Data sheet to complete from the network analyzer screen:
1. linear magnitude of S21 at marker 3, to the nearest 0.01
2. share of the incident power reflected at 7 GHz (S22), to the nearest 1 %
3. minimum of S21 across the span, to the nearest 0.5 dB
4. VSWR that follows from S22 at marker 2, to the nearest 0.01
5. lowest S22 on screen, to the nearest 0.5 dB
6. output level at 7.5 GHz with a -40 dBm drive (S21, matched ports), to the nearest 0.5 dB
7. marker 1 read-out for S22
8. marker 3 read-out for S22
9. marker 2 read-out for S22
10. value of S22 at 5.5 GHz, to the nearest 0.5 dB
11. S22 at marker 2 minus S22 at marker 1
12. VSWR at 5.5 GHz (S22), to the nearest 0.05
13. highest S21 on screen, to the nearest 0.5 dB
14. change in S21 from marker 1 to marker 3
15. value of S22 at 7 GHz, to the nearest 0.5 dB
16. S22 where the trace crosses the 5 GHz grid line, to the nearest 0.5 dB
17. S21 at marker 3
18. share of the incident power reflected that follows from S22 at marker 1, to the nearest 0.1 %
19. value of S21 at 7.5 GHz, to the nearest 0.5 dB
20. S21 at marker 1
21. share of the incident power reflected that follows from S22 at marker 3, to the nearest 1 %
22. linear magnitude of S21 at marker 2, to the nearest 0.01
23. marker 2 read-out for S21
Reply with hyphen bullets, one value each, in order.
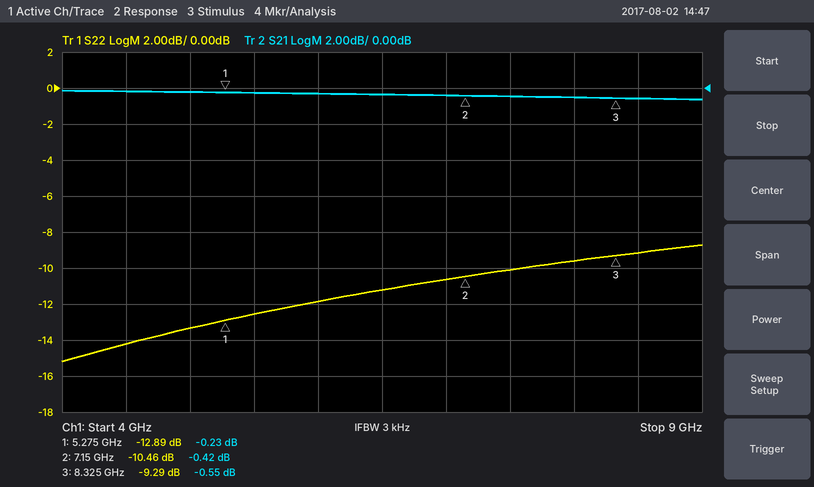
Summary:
- 0.94
- 9 %
- -0.5 dB
- 1.86
- -15.0 dB
- -40.5 dBm
- -12.89 dB
- -9.29 dB
- -10.46 dB
- -12.5 dB
- 2.43 dB
- 1.60
- 0.0 dB
- -0.32 dB
- -10.5 dB
- -13.5 dB
- -0.55 dB
- 5.1 %
- -0.5 dB
- -0.23 dB
- 12 %
- 0.95
- -0.42 dB
